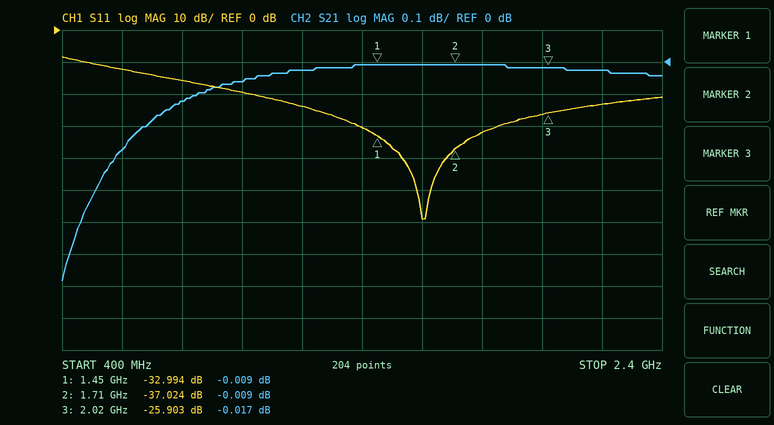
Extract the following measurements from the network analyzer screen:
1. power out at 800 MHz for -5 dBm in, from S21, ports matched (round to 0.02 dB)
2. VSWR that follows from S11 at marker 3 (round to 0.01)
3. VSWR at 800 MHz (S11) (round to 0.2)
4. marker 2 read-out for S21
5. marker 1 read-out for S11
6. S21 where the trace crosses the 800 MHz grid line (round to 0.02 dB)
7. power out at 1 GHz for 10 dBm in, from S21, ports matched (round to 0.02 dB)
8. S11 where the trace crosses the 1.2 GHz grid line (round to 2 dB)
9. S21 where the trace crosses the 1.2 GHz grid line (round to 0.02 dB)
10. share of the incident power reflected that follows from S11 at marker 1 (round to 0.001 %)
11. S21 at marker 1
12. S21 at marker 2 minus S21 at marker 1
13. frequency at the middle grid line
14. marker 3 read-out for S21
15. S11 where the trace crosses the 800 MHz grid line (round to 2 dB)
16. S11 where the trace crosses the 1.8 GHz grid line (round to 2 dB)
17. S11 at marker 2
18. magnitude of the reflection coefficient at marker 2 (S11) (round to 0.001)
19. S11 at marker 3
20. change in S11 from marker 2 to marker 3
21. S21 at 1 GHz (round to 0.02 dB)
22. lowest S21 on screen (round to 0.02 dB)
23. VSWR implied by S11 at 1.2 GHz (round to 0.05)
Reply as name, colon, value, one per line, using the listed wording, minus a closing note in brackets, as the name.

power out at 800 MHz for -5 dBm in, from S21, ports matched: -5.12 dBm
VSWR that follows from S11 at marker 3: 1.11
VSWR at 800 MHz (S11): 1.4
marker 2 read-out for S21: -0.009 dB
marker 1 read-out for S11: -32.994 dB
S21 where the trace crosses the 800 MHz grid line: -0.12 dB
power out at 1 GHz for 10 dBm in, from S21, ports matched: 9.94 dBm
S11 where the trace crosses the 1.2 GHz grid line: -24 dB
S21 where the trace crosses the 1.2 GHz grid line: -0.02 dB
share of the incident power reflected that follows from S11 at marker 1: 0.050 %
S21 at marker 1: -0.009 dB
S21 at marker 2 minus S21 at marker 1: 0.000 dB
frequency at the middle grid line: 1.4 GHz
marker 3 read-out for S21: -0.017 dB
S11 where the trace crosses the 800 MHz grid line: -16 dB
S11 where the trace crosses the 1.8 GHz grid line: -32 dB
S11 at marker 2: -37.024 dB
magnitude of the reflection coefficient at marker 2 (S11): 0.014
S11 at marker 3: -25.903 dB
change in S11 from marker 2 to marker 3: 11.121 dB
S21 at 1 GHz: -0.06 dB
lowest S21 on screen: -0.68 dB
VSWR implied by S11 at 1.2 GHz: 1.15
